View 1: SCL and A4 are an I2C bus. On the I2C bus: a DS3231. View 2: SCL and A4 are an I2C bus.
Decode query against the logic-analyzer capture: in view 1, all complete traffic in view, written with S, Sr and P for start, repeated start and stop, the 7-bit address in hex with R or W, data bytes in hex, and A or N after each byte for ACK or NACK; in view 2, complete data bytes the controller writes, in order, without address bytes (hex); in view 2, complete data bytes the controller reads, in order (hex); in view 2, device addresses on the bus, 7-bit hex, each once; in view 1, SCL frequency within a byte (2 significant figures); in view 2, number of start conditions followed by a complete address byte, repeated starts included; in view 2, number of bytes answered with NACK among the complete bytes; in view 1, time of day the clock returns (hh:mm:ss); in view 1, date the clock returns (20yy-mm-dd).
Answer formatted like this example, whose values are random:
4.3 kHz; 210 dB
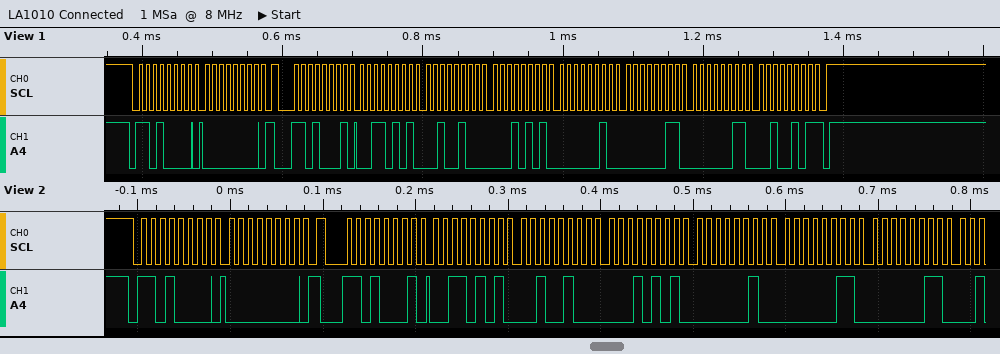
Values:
S 68W A 00 A Sr 68R A 35 A 24 A 15 A 02 A 03 A 03 A 25 N P; 00; 35 24 15 02 03 03; 0x68; 100 kHz; 2; 0; 15:24:35; 2025-03-03
